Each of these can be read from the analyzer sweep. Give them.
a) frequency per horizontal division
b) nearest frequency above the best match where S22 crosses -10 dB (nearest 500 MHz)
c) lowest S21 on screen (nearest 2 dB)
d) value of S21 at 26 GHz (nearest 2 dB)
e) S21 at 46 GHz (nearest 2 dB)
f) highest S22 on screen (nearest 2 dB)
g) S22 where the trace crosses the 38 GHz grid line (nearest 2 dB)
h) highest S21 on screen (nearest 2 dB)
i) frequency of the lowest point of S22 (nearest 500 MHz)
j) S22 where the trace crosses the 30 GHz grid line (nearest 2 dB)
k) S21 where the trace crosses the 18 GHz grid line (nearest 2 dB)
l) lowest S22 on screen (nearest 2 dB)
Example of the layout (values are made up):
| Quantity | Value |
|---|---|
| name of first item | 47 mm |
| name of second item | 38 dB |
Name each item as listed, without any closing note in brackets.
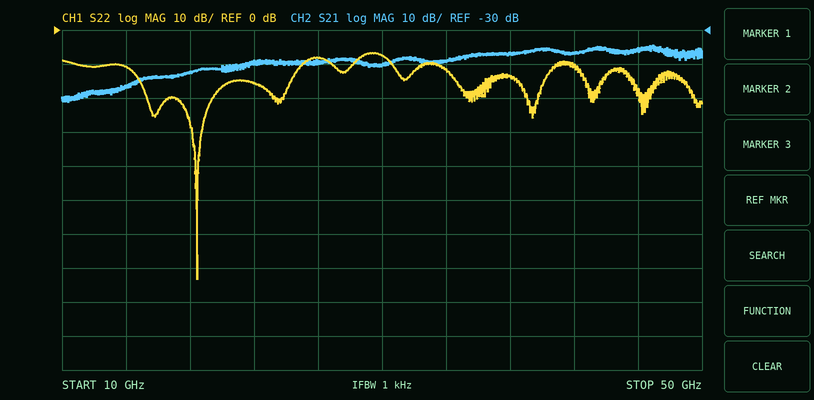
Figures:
| Quantity | Value |
|---|---|
| frequency per horizontal division | 4 GHz |
| nearest frequency above the best match where S22 crosses -10 dB | 25.0 GHz |
| lowest S21 on screen | -52 dB |
| value of S21 at 26 GHz | -40 dB |
| S21 at 46 GHz | -36 dB |
| highest S22 on screen | -6 dB |
| S22 where the trace crosses the 38 GHz grid line | -14 dB |
| highest S21 on screen | -34 dB |
| frequency of the lowest point of S22 | 18.5 GHz |
| S22 where the trace crosses the 30 GHz grid line | -8 dB |
| S21 where the trace crosses the 18 GHz grid line | -42 dB |
| lowest S22 on screen | -74 dB |
